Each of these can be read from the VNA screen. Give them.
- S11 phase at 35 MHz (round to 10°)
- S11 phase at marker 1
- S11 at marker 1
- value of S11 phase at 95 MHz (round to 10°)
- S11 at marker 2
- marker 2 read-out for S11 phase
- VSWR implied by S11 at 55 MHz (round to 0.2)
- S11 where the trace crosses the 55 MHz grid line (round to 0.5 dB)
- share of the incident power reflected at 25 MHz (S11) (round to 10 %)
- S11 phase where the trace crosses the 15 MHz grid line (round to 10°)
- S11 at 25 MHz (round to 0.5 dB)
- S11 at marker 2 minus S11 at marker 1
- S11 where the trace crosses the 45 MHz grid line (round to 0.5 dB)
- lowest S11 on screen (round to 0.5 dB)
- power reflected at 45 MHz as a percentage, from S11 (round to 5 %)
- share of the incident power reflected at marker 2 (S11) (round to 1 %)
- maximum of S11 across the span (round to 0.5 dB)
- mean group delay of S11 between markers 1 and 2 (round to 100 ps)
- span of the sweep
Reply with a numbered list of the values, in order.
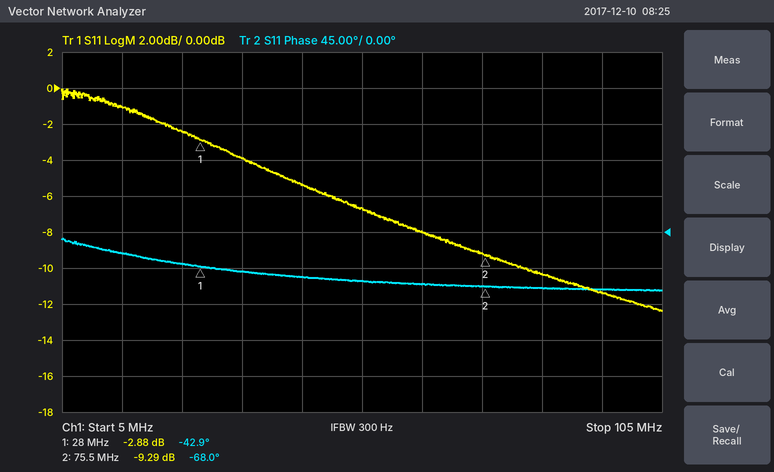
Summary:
1. -50°
2. -42.9°
3. -2.88 dB
4. -70°
5. -9.29 dB
6. -68.0°
7. 2.8
8. -6.5 dB
9. 60 %
10. -30°
11. -2.5 dB
12. -6.41 dB
13. -5.5 dB
14. -12.5 dB
15. 30 %
16. 12 %
17. 0.0 dB
18. 1.5 ns
19. 100 MHz
